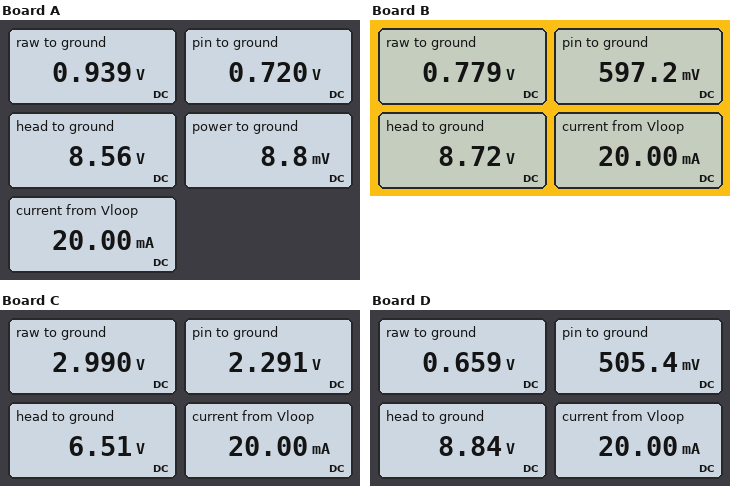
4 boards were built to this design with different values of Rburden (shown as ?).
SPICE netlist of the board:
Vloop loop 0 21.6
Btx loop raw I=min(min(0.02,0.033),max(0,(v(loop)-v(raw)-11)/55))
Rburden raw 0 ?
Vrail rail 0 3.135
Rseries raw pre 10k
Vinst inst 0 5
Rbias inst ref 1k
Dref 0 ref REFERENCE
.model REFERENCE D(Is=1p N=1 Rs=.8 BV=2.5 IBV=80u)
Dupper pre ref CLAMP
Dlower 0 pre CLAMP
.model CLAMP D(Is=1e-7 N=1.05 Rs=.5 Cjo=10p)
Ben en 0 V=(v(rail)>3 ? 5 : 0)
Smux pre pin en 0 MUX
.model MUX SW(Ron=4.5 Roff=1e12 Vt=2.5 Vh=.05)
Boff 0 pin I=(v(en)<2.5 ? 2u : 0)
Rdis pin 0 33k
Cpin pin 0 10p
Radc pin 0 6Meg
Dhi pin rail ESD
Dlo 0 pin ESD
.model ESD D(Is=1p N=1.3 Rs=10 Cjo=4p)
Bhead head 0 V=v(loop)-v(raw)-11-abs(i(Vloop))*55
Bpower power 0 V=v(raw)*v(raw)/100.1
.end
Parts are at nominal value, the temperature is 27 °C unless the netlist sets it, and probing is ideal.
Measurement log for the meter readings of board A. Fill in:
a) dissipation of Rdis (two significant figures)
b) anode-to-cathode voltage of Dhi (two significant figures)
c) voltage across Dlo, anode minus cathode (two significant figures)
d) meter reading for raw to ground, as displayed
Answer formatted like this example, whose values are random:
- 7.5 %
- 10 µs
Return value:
- 16 µW
- -2.4 V
- -720 mV
- 0.939 V
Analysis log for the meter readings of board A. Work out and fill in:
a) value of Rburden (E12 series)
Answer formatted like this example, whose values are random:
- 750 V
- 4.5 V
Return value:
- 47 Ω
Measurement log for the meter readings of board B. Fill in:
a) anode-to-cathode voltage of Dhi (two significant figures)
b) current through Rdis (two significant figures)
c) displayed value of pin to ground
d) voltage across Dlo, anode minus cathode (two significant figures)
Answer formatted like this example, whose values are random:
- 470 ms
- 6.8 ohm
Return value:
- -2.5 V
- 18 µA
- 597.2 mV
- -600 mV
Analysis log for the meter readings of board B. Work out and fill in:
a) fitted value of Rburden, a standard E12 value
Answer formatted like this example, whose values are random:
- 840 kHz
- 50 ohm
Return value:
- 39 Ω
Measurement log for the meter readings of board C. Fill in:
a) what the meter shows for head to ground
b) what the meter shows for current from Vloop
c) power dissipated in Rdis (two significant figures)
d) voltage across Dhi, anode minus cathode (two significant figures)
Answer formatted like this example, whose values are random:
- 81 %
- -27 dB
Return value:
- 6.51 V
- 20.00 mA
- 160 µW
- -840 mV
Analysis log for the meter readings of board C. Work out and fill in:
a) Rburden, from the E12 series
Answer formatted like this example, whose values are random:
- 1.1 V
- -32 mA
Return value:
- 150 Ω
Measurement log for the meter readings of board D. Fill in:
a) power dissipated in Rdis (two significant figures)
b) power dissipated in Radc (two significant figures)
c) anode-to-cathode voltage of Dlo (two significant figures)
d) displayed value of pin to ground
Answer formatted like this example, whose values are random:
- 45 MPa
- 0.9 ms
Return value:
- 7.7 µW
- 43 nW
- -510 mV
- 505.4 mV
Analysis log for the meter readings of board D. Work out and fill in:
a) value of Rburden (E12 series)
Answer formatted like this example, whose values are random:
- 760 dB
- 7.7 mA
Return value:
- 33 Ω
